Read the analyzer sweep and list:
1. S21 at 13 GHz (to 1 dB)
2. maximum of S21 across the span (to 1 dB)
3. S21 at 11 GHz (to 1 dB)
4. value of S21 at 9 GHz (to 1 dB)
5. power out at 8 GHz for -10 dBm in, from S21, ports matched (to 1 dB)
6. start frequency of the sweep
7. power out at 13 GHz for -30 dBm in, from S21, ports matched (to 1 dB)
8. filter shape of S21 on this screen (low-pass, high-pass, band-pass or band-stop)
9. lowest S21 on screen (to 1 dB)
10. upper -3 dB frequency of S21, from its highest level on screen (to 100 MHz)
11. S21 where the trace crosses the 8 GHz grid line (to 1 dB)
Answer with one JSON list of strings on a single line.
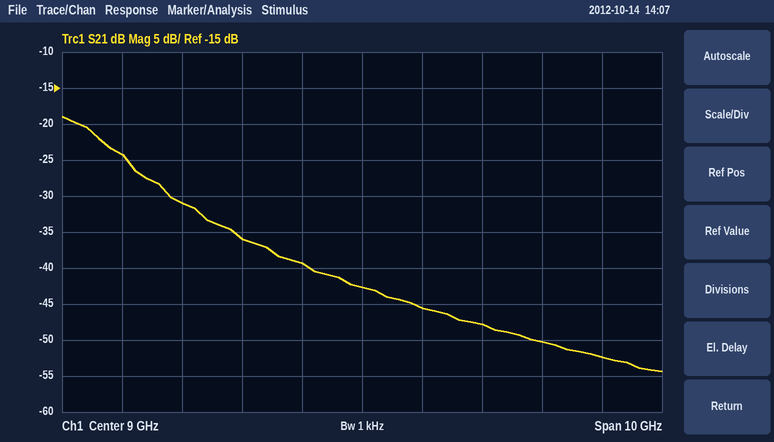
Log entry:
["-52 dB", "-19 dB", "-48 dB", "-43 dB", "-49 dBm", "4 GHz", "-82 dBm", "low-pass", "-54 dB", "4.6 GHz", "-39 dB"]
